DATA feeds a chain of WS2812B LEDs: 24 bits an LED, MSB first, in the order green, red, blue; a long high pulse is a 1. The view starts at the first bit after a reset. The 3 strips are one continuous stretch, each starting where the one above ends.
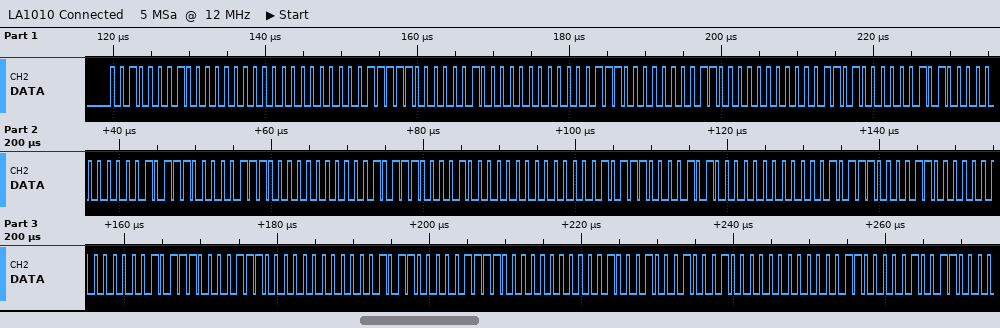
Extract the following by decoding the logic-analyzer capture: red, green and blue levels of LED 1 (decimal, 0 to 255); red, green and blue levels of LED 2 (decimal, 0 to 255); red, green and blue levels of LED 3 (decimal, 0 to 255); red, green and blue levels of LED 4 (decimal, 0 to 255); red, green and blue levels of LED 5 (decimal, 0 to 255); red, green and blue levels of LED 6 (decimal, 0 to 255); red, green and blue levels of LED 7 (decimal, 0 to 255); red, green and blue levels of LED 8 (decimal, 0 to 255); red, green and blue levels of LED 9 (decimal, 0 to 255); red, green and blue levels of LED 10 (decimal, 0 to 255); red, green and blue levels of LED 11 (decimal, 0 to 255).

0, 33, 0
2, 31, 0
3, 28, 0
5, 26, 0
7, 23, 0
8, 23, 0
10, 23, 0
12, 23, 0
14, 23, 0
15, 22, 0
17, 17, 0
